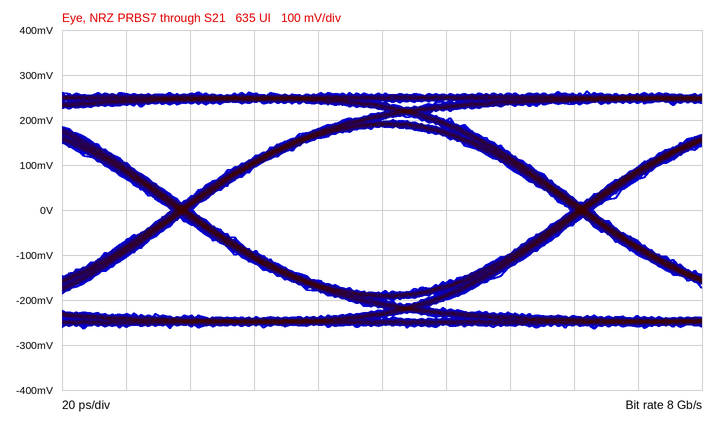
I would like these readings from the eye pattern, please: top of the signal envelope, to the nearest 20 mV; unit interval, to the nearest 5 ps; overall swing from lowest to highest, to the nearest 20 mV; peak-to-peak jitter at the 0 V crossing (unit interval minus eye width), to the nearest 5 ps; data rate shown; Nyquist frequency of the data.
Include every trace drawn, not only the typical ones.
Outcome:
260 mV
125 ps
520 mV
5 ps
8 Gb/s
4 GHz
